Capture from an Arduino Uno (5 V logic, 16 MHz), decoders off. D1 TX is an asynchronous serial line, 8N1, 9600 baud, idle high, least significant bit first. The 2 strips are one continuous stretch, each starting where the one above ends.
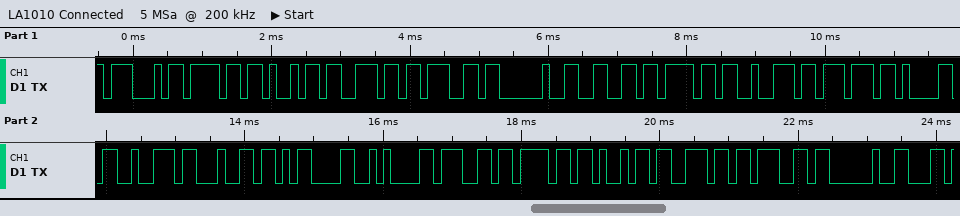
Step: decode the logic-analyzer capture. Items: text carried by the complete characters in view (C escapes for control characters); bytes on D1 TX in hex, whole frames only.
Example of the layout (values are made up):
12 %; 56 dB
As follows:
"Going forward\r\ngoing "; 47 6F 69 6E 67 20 66 6F 72 77 61 72 64 0D 0A 67 6F 69 6E 67 20
